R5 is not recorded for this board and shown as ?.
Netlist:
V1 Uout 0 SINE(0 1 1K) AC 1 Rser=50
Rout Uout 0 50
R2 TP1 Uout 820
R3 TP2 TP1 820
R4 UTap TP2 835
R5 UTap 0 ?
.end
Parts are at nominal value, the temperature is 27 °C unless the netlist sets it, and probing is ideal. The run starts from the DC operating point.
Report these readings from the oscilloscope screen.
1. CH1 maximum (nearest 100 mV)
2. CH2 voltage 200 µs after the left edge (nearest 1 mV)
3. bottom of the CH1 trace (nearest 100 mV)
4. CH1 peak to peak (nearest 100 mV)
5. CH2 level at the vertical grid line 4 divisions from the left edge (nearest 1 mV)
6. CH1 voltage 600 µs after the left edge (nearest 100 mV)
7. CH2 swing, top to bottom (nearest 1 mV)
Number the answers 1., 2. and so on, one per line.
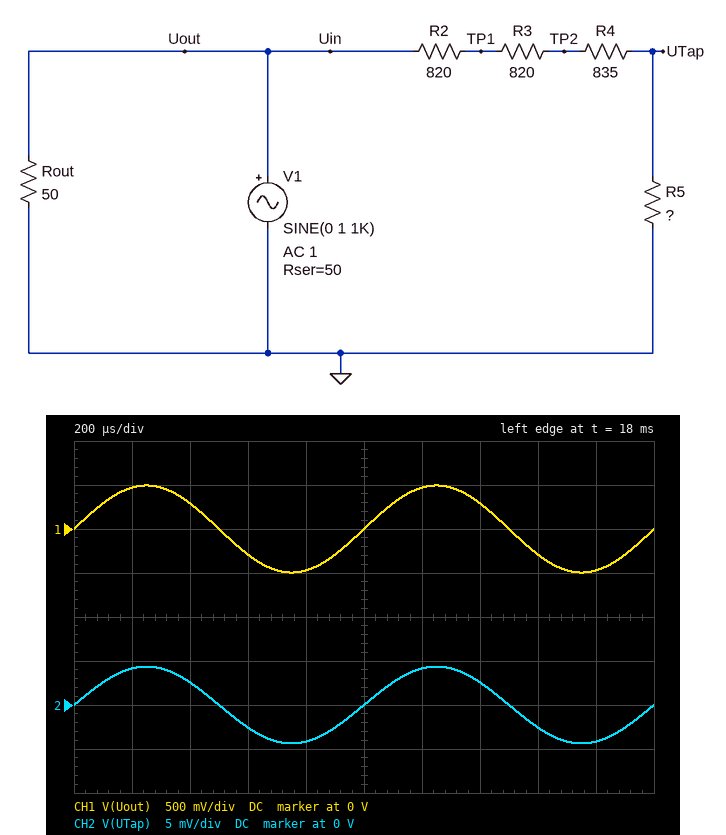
1. 500 mV
2. 4 mV
3. -500 mV
4. 1.0 V
5. -4 mV
6. -300 mV
7. 9 mV
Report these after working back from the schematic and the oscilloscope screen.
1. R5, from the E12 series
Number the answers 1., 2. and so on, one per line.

1. 22 Ω
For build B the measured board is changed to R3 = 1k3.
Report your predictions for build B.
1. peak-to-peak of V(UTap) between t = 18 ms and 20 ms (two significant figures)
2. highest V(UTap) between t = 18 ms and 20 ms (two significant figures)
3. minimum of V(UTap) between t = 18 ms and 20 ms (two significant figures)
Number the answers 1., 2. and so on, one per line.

1. 7.3 mV
2. 3.7 mV
3. -3.7 mV
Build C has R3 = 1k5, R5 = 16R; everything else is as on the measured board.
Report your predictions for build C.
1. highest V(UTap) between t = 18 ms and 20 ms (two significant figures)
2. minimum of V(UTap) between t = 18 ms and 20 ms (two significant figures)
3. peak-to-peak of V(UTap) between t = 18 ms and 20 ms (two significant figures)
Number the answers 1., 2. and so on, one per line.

1. 2.5 mV
2. -2.5 mV
3. 5.0 mV
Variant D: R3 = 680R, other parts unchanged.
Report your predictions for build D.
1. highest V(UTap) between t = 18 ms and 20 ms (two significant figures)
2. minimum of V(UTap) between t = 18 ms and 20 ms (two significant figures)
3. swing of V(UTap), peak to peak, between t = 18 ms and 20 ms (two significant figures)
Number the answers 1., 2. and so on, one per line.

1. 4.6 mV
2. -4.6 mV
3. 9.2 mV
